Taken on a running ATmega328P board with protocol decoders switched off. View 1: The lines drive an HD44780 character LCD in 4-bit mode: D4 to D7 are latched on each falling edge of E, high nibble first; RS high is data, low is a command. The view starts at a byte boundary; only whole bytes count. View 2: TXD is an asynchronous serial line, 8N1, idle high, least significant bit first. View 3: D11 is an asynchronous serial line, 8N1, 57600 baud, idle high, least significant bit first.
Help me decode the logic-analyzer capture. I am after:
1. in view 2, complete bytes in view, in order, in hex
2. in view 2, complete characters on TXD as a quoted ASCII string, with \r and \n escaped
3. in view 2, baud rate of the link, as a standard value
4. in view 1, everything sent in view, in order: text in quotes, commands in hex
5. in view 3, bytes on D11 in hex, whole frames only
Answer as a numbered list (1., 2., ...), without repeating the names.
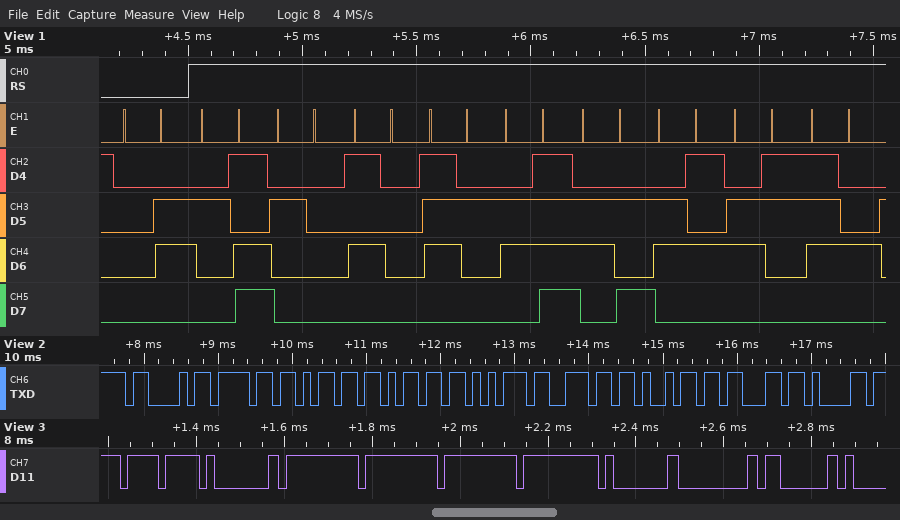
1. 43 6F 6D 6D 75 6E 69 63 61
2. "Communica"
3. 9600 baud
4. 0x06 "- Project"
5. 0xEF 0x01 0xFF 0xFF 0xFF 0xFF 0x01 0x00 0x03
